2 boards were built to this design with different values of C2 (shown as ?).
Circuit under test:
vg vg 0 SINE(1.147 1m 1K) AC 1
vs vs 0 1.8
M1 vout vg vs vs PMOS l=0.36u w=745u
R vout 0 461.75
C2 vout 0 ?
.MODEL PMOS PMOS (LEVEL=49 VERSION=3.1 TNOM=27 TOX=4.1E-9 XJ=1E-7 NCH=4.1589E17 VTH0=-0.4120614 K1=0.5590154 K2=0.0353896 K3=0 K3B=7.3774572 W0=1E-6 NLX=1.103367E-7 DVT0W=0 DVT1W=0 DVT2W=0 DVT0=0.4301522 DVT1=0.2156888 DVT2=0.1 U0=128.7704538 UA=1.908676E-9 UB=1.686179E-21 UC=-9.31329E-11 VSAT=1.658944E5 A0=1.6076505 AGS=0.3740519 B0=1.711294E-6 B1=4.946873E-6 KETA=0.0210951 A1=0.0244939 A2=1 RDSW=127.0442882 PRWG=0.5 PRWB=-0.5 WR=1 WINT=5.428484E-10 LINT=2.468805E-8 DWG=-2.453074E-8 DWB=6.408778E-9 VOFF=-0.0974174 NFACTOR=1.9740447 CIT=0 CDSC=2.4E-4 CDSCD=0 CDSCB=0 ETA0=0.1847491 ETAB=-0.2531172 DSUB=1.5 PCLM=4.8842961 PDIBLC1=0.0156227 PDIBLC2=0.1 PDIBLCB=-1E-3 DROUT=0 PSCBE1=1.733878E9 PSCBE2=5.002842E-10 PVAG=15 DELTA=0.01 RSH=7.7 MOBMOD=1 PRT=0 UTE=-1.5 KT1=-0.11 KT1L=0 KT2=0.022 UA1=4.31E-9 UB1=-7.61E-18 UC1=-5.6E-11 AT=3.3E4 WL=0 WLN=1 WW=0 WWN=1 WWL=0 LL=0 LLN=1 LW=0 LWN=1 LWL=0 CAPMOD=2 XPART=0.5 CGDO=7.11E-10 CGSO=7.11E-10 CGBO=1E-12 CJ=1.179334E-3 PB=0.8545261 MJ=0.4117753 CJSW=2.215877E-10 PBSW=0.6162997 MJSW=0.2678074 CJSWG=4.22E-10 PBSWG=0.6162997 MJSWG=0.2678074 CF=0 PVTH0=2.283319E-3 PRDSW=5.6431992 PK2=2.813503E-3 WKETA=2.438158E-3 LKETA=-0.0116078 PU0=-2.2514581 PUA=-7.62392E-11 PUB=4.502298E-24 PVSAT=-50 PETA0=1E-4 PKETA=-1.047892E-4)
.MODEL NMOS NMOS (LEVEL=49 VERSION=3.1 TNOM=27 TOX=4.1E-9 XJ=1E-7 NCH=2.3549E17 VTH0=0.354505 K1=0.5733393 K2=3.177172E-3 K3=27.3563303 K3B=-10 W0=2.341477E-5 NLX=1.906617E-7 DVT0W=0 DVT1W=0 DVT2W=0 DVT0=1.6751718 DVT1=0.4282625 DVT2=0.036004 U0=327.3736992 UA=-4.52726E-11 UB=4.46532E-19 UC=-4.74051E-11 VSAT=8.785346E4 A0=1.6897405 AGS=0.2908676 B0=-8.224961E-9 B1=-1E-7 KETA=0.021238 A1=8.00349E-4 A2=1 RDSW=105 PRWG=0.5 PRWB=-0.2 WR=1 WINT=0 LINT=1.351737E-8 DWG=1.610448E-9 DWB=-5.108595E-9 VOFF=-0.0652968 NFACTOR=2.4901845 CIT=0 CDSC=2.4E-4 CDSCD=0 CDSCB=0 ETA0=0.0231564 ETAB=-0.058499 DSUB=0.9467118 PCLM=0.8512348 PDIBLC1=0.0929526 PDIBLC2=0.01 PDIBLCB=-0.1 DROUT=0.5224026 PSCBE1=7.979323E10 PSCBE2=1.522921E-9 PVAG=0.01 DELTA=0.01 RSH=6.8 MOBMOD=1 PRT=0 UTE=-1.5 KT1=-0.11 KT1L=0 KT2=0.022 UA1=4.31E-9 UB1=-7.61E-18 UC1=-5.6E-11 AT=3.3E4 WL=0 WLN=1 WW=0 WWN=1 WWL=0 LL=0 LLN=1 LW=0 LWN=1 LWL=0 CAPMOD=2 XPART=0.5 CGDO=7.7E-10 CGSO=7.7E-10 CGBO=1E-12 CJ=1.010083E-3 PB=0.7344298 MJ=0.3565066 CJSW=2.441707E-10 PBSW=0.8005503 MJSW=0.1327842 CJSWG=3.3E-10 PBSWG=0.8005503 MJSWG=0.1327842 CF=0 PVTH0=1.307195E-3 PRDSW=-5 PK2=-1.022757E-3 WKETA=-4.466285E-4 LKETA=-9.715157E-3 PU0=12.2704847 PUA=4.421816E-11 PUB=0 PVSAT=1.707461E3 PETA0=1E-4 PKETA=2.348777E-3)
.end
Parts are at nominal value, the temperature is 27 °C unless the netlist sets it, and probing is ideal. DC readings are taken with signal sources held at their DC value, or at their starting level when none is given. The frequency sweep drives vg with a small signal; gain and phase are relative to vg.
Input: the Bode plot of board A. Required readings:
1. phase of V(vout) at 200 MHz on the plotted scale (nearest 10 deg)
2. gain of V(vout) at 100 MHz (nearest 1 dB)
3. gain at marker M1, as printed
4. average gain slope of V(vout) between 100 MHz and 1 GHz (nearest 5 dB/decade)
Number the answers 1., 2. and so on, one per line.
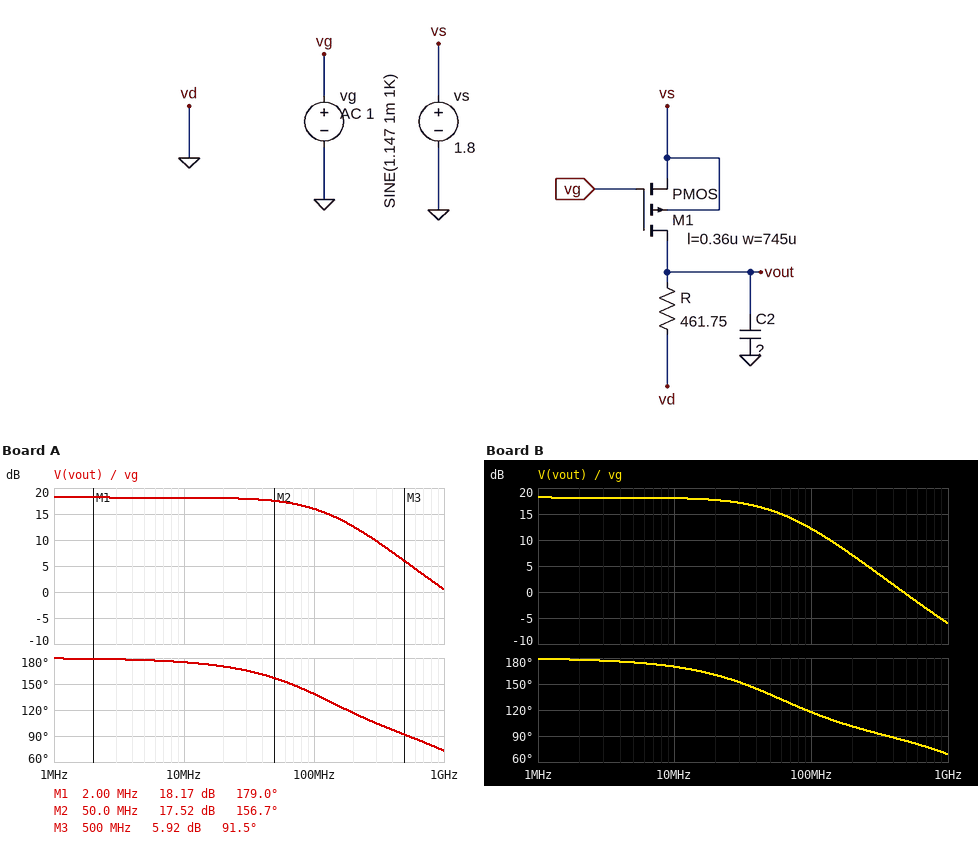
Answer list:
1. 120 deg
2. 16 dB
3. 18.17 dB
4. -15 dB/decade
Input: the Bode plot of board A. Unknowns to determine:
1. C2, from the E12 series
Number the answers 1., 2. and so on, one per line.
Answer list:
1. 2.2 pF
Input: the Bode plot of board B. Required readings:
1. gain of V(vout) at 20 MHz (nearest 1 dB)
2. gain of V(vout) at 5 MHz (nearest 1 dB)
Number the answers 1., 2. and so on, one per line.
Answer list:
1. 18 dB
2. 18 dB
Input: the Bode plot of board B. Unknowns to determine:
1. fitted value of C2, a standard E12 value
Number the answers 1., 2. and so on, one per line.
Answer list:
1. 5.6 pF
